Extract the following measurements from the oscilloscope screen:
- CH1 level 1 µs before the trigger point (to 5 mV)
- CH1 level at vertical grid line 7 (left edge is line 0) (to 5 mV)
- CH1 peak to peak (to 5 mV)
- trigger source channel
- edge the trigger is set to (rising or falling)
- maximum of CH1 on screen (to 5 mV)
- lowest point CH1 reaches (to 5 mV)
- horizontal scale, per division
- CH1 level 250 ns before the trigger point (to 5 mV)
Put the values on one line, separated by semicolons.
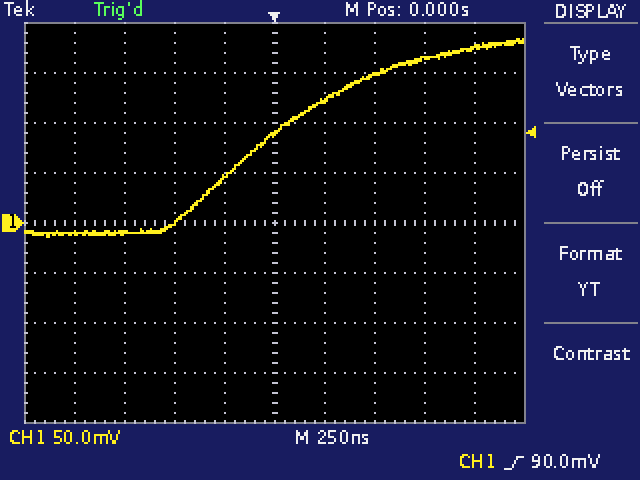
-10 mV; 150 mV; 200 mV; CH1; rising; 185 mV; -15 mV; 250 ns; 45 mV
